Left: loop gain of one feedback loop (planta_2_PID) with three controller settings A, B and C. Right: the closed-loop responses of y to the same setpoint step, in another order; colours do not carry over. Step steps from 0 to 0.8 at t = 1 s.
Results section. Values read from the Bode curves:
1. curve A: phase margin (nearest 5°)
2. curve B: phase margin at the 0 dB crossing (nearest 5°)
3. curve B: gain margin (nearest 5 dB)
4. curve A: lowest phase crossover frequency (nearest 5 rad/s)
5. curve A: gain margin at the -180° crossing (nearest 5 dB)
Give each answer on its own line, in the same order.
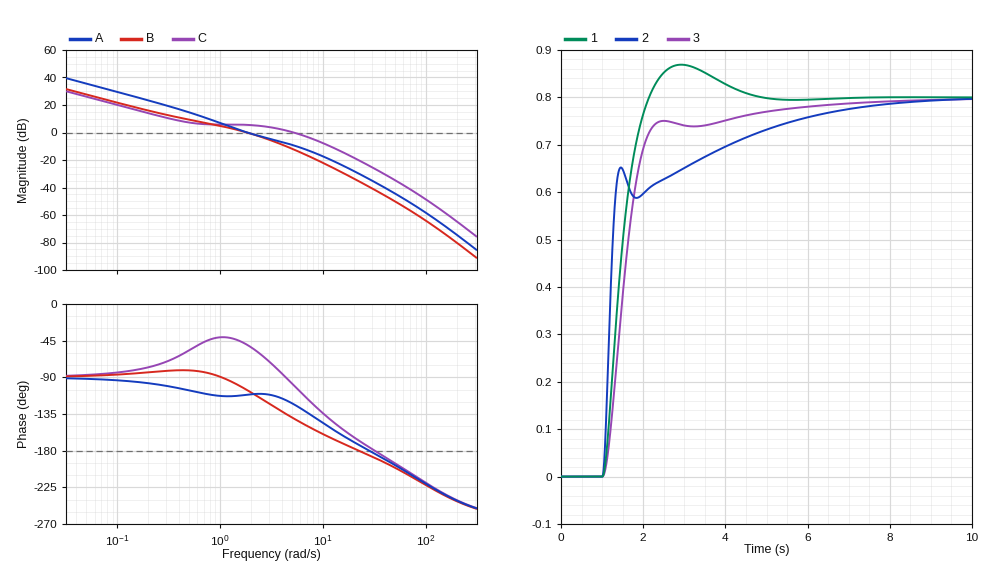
70°
75°
35 dB
30 rad/s
35 dB
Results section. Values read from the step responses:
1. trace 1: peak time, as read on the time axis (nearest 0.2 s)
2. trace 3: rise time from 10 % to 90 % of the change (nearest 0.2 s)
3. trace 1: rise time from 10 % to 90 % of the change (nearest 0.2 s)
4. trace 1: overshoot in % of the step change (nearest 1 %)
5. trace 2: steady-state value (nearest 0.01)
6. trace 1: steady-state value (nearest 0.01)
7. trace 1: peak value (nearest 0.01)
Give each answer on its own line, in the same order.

3.0 s
1.0 s
0.8 s
9 %
0.80
0.80
0.87
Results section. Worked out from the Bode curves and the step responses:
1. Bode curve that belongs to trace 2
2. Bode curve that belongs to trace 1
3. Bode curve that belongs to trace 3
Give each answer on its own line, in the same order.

C
A
B
